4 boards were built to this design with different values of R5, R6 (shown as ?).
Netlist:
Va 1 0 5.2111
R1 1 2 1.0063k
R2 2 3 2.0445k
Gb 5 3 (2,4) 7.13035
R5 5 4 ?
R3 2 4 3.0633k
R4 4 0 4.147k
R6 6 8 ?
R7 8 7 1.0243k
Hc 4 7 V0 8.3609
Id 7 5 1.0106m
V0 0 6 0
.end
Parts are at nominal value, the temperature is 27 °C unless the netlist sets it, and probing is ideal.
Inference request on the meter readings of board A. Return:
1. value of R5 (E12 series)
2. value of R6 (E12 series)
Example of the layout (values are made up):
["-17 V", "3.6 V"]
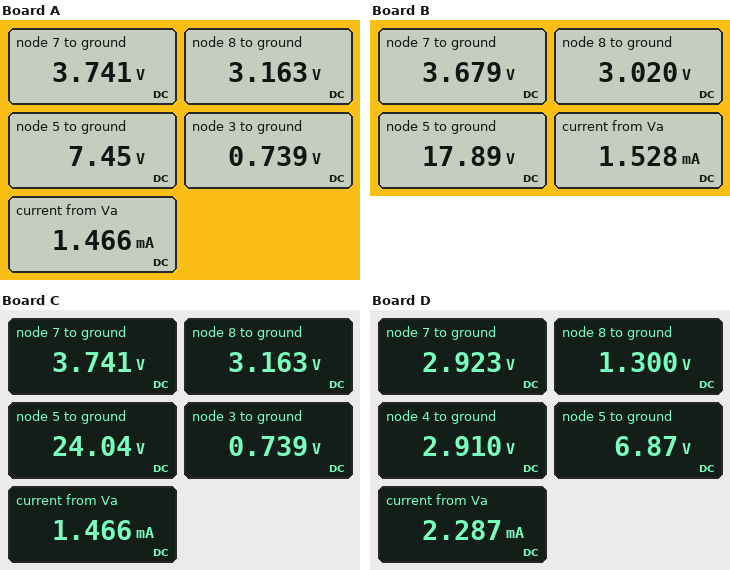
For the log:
["1.5 kΩ", "5.6 kΩ"]
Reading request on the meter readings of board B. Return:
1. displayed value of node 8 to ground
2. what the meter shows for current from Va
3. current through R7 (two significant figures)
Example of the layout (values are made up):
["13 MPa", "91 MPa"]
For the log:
["3.020 V", "1.528 mA", "640 µA"]
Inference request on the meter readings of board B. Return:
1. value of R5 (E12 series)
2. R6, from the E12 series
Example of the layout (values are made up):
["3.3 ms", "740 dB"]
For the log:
["5.6 kΩ", "4.7 kΩ"]
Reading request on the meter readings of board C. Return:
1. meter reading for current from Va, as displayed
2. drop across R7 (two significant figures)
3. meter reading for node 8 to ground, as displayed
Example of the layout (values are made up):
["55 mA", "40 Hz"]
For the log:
["1.466 mA", "580 mV", "3.163 V"]
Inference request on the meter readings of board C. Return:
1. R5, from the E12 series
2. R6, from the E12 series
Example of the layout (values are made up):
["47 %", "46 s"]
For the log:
["8.2 kΩ", "5.6 kΩ"]
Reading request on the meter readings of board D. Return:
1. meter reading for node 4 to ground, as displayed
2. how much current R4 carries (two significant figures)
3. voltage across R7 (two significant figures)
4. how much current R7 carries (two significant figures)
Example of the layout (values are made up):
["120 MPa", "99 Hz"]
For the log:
["2.910 V", "700 µA", "1.6 V", "1.6 mA"]
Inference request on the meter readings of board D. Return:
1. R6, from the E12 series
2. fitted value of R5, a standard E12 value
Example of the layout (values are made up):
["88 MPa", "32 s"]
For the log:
["820 Ω", "1.2 kΩ"]
